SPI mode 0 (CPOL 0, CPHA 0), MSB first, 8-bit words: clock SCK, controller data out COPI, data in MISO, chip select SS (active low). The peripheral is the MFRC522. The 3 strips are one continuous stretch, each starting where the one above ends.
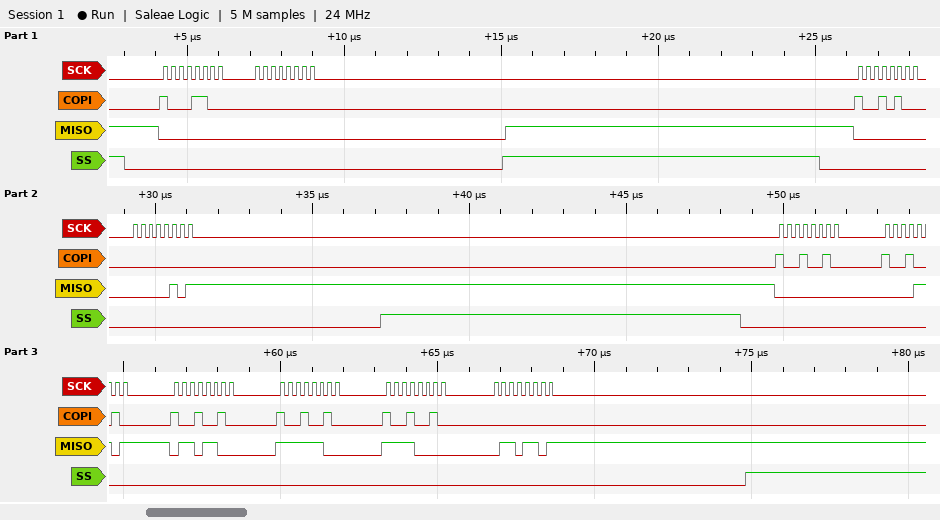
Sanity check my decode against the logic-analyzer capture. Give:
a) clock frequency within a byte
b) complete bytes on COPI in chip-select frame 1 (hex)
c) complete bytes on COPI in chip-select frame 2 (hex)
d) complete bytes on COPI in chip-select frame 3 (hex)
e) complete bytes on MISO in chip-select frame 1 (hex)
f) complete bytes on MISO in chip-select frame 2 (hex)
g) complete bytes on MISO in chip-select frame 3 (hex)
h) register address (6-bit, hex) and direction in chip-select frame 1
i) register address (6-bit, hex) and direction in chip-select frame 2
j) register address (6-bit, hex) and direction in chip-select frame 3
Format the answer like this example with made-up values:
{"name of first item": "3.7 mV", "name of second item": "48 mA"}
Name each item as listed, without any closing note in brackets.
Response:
{"clock frequency within a byte": "4 MHz", "complete bytes on COPI in chip-select frame 1": "8C 00", "complete bytes on COPI in chip-select frame 2": "94 00", "complete bytes on COPI in chip-select frame 3": "92 92 92 92 92 00", "complete bytes on MISO in chip-select frame 1": "00 00", "complete bytes on MISO in chip-select frame 2": "00 05", "complete bytes on MISO in chip-select frame 3": "00 0D 6C FC F0 6D", "register address (6-bit, hex) and direction in chip-select frame 1": "0x06 read", "register address (6-bit, hex) and direction in chip-select frame 2": "0x0A read", "register address (6-bit, hex) and direction in chip-select frame 3": "0x09 read"}
